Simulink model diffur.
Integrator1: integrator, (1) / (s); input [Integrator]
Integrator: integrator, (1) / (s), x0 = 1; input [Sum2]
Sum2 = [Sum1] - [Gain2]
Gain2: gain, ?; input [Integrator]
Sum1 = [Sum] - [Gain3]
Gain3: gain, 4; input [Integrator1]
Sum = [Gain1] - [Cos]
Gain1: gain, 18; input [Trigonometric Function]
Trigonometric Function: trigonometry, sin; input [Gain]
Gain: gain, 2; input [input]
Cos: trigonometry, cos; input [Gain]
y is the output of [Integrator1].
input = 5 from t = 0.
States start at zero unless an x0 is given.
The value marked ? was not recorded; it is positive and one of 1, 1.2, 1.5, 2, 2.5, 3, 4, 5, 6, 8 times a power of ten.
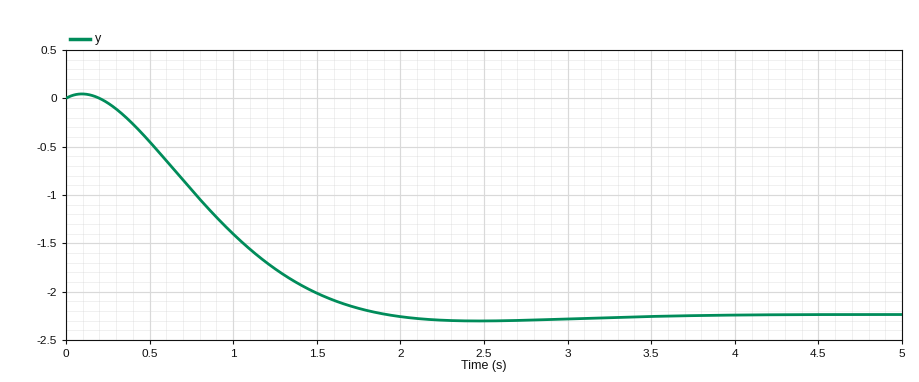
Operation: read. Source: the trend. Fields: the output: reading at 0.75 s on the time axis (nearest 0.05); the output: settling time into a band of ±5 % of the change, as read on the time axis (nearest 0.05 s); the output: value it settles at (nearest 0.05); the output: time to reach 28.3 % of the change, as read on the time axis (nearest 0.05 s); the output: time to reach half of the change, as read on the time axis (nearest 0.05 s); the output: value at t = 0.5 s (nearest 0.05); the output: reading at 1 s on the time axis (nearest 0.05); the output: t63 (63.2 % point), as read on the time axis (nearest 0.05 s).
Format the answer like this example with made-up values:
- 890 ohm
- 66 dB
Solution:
- -0.95
- 1.65 s
- -2.25
- 0.60 s
- 0.85 s
- -0.45
- -1.40
- 1.00 s
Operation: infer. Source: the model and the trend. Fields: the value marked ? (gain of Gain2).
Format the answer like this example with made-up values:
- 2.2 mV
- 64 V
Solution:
- 3
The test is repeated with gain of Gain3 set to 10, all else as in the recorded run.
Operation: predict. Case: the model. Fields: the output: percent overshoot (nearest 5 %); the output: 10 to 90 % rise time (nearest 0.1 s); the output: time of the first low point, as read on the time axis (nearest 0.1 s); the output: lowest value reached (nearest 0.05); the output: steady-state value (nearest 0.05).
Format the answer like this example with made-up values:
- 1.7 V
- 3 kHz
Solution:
- 20 %
- 0.5 s
- 1.2 s
- -1.05
- -0.90
